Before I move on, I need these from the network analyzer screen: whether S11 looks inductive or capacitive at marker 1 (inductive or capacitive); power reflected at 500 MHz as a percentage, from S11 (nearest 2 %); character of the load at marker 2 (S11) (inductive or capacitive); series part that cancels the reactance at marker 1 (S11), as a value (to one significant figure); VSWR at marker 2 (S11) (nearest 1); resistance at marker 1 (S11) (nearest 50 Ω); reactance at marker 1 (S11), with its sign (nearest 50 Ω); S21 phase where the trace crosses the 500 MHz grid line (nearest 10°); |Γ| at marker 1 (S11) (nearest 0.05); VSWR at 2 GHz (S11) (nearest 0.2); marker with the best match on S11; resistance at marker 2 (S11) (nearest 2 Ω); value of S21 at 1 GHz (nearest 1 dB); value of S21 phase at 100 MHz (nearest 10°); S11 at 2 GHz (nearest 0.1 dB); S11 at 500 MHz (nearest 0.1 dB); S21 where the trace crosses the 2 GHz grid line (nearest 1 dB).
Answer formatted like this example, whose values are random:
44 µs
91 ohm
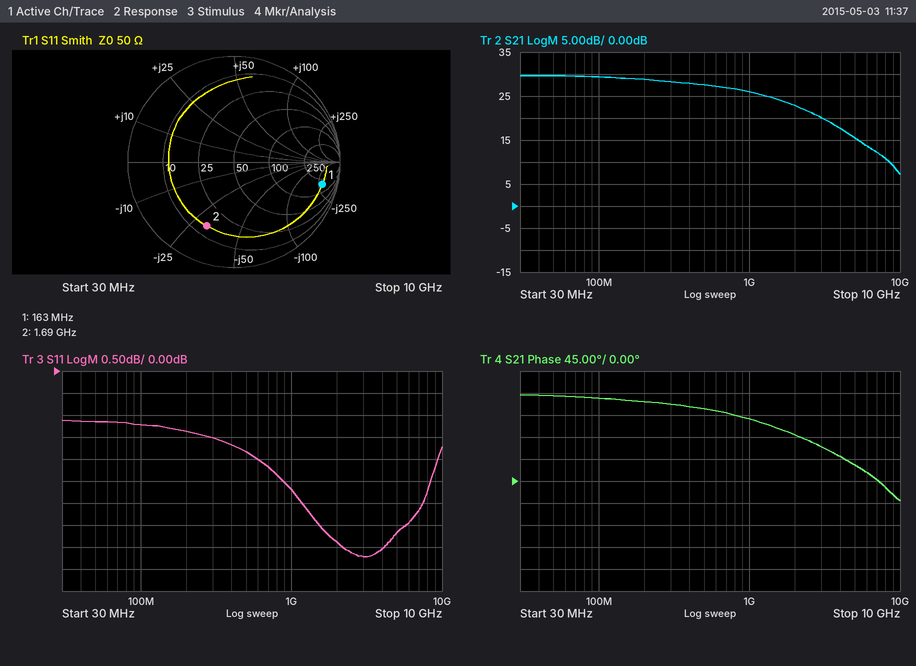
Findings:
capacitive
66 %
capacitive
300 nH
5
200 Ω
-300 Ω
150°
0.85
4.6
marker 2
14 Ω
26 dB
170°
-3.9 dB
-1.8 dB
23 dB
